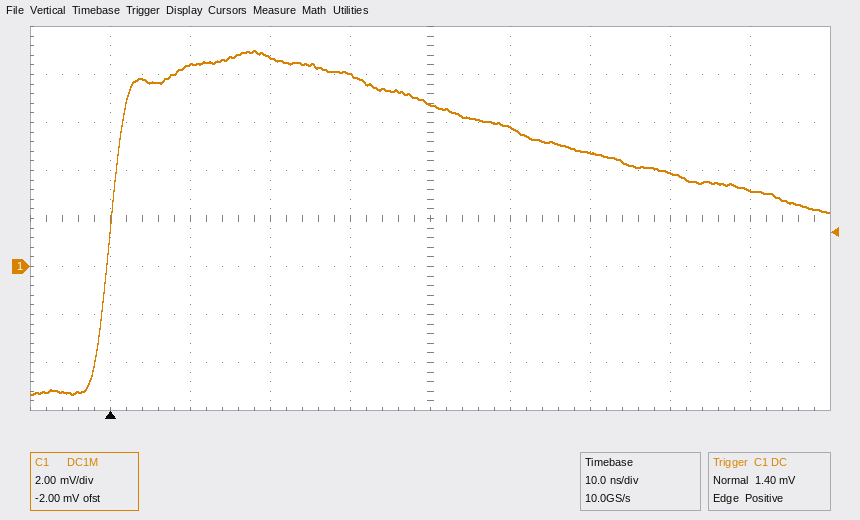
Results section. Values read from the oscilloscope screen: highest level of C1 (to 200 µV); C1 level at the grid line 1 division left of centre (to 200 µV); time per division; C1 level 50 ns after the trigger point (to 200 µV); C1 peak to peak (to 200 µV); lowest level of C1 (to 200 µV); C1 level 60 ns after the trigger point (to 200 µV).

9.0 mV
8.0 mV
10 ns
5.8 mV
14.4 mV
-5.4 mV
4.8 mV
